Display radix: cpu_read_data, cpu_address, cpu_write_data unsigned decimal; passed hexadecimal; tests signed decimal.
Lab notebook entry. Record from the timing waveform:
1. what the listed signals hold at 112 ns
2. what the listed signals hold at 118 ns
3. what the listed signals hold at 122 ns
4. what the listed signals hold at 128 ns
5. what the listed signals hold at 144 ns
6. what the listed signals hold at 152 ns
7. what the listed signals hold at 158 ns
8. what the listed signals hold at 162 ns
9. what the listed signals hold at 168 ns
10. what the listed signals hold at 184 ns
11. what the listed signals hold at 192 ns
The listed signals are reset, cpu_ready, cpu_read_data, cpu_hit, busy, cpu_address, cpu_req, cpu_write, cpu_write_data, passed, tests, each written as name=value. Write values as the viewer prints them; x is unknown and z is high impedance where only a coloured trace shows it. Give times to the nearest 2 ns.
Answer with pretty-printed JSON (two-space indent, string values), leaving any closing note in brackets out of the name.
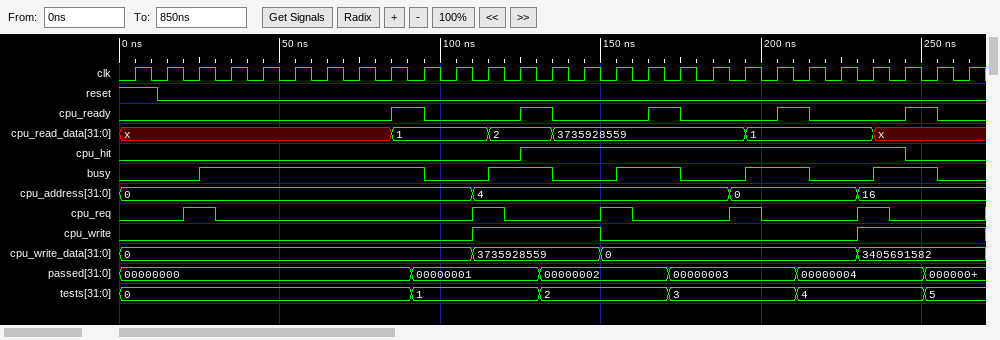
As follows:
{
  "what the listed signals hold at 112 ns": "reset=0, cpu_ready=0, cpu_read_data=1, cpu_hit=0, busy=0, cpu_address=4, cpu_req=1, cpu_write=1, cpu_write_data=3735928559, passed=00000001, tests=1",
  "what the listed signals hold at 118 ns": "reset=0, cpu_ready=0, cpu_read_data=2, cpu_hit=0, busy=1, cpu_address=4, cpu_req=1, cpu_write=1, cpu_write_data=3735928559, passed=00000001, tests=1",
  "what the listed signals hold at 122 ns": "reset=0, cpu_ready=0, cpu_read_data=2, cpu_hit=0, busy=1, cpu_address=4, cpu_req=0, cpu_write=1, cpu_write_data=3735928559, passed=00000001, tests=1",
  "what the listed signals hold at 128 ns": "reset=0, cpu_ready=1, cpu_read_data=2, cpu_hit=1, busy=1, cpu_address=4, cpu_req=0, cpu_write=1, cpu_write_data=3735928559, passed=00000001, tests=1",
  "what the listed signals hold at 144 ns": "reset=0, cpu_ready=0, cpu_read_data=3735928559, cpu_hit=1, busy=0, cpu_address=4, cpu_req=0, cpu_write=1, cpu_write_data=3735928559, passed=00000002, tests=2",
  "what the listed signals hold at 152 ns": "reset=0, cpu_ready=0, cpu_read_data=3735928559, cpu_hit=1, busy=0, cpu_address=4, cpu_req=1, cpu_write=0, cpu_write_data=0, passed=00000002, tests=2",
  "what the listed signals hold at 158 ns": "reset=0, cpu_ready=0, cpu_read_data=3735928559, cpu_hit=1, busy=1, cpu_address=4, cpu_req=1, cpu_write=0, cpu_write_data=0, passed=00000002, tests=2",
  "what the listed signals hold at 162 ns": "reset=0, cpu_ready=0, cpu_read_data=3735928559, cpu_hit=1, busy=1, cpu_address=4, cpu_req=0, cpu_write=0, cpu_write_data=0, passed=00000002, tests=2",
  "what the listed signals hold at 168 ns": "reset=0, cpu_ready=1, cpu_read_data=3735928559, cpu_hit=1, busy=1, cpu_address=4, cpu_req=0, cpu_write=0, cpu_write_data=0, passed=00000002, tests=2",
  "what the listed signals hold at 184 ns": "reset=0, cpu_ready=0, cpu_read_data=3735928559, cpu_hit=1, busy=0, cpu_address=4, cpu_req=0, cpu_write=0, cpu_write_data=0, passed=00000003, tests=3",
  "what the listed signals hold at 192 ns": "reset=0, cpu_ready=0, cpu_read_data=3735928559, cpu_hit=1, busy=0, cpu_address=0, cpu_req=1, cpu_write=0, cpu_write_data=0, passed=00000003, tests=3"
}
